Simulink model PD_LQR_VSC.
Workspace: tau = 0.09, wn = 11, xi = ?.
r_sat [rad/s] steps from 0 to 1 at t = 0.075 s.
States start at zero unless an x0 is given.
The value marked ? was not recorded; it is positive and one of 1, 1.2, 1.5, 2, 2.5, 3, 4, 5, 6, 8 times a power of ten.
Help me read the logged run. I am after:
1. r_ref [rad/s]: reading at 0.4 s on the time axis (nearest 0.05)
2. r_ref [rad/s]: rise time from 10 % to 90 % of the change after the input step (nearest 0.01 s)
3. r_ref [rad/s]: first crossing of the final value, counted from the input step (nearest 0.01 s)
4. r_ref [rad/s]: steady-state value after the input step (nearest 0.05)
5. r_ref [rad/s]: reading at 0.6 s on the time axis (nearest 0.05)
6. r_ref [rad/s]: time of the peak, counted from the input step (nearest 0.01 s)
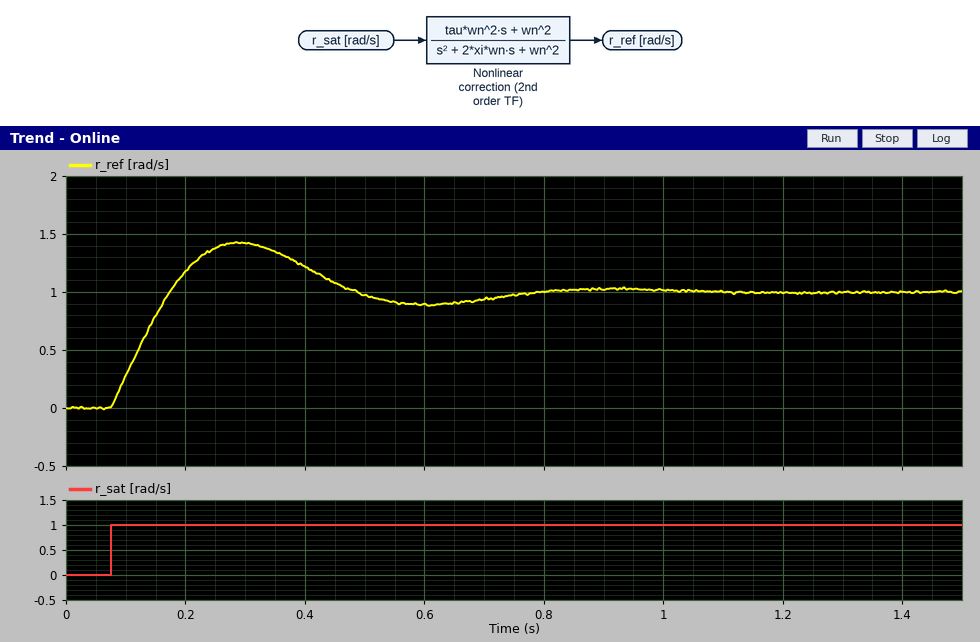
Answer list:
1.20
0.08 s
0.10 s
1.00
0.90
0.21 s
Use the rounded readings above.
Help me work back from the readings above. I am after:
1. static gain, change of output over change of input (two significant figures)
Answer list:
1.0
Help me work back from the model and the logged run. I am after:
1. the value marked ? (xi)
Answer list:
0.4
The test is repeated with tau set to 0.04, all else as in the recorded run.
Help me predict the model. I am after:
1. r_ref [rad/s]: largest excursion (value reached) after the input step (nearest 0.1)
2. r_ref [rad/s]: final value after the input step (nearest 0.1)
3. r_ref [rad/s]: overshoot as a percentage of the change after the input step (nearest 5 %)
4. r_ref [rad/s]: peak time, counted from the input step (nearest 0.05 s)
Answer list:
1.3
1.0
30 %
0.25 s
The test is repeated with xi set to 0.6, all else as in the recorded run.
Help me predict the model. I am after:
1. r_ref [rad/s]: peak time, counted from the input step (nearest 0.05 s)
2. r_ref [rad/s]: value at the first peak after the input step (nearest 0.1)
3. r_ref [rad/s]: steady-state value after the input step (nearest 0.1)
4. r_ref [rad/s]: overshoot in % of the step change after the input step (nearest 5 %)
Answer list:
0.25 s
1.2
1.0
20 %
